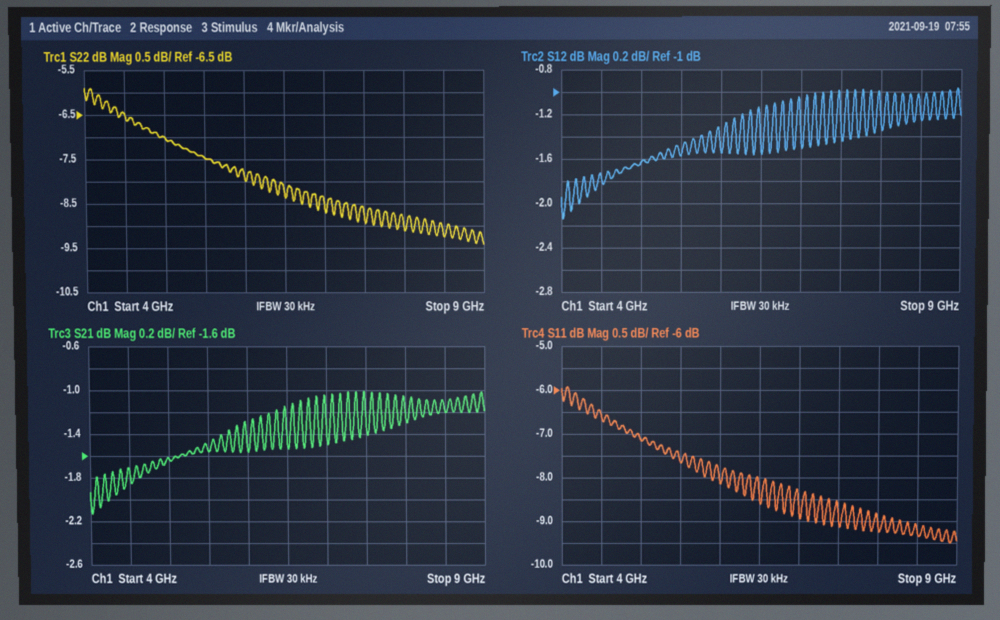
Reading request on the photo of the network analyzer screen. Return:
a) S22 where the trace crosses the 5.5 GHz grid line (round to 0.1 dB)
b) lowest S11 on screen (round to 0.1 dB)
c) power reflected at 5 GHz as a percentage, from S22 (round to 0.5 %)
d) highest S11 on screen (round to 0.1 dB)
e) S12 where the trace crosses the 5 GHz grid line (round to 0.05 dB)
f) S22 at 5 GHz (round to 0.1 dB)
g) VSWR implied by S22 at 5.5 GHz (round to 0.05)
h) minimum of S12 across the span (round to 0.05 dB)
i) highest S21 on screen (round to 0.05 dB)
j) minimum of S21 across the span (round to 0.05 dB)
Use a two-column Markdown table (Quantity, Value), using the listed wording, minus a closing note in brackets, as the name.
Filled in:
| Quantity | Value |
|---|---|
| S22 where the trace crosses the 5.5 GHz grid line | -7.5 dB |
| lowest S11 on screen | -9.5 dB |
| power reflected at 5 GHz as a percentage, from S22 | 20.0 % |
| highest S11 on screen | -5.9 dB |
| S12 where the trace crosses the 5 GHz grid line | -1.65 dB |
| S22 at 5 GHz | -7.0 dB |
| VSWR implied by S22 at 5.5 GHz | 2.45 |
| minimum of S12 across the span | -2.15 dB |
| highest S21 on screen | -1.00 dB |
| minimum of S21 across the span | -2.15 dB |
